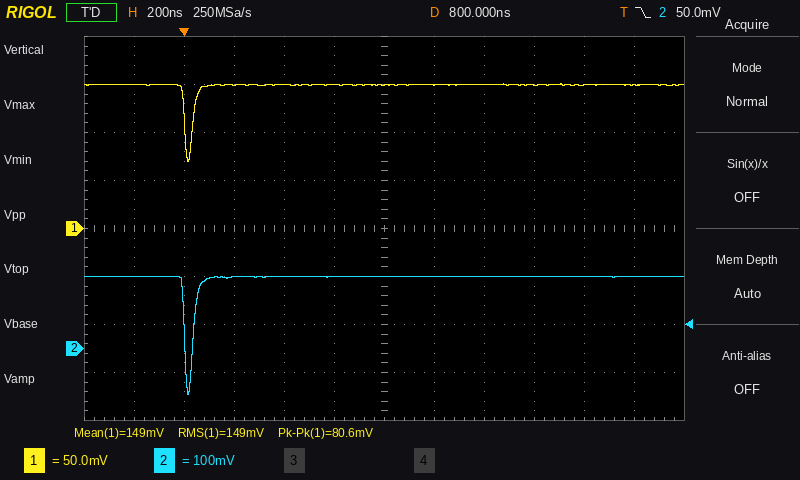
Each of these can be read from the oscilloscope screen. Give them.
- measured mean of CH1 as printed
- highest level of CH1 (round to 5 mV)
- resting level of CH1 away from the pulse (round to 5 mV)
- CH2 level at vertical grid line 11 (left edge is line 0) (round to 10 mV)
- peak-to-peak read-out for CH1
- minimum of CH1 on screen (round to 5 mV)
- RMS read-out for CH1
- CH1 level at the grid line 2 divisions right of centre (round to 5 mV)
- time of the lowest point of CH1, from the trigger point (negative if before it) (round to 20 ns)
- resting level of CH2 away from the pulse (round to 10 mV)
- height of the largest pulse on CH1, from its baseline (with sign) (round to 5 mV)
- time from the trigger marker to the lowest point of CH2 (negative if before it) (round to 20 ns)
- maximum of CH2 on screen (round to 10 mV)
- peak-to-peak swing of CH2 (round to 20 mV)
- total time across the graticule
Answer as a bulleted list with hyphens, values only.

- 149 mV
- 150 mV
- 150 mV
- 150 mV
- 80.6 mV
- 70 mV
- 149 mV
- 150 mV
- +20 ns
- 150 mV
- -80 mV
- +20 ns
- 150 mV
- 240 mV
- 2.4 µs
